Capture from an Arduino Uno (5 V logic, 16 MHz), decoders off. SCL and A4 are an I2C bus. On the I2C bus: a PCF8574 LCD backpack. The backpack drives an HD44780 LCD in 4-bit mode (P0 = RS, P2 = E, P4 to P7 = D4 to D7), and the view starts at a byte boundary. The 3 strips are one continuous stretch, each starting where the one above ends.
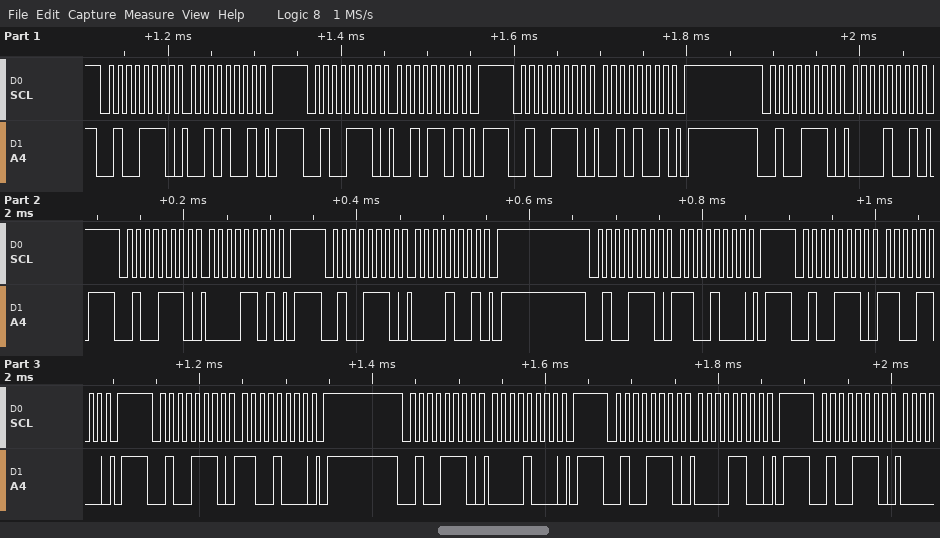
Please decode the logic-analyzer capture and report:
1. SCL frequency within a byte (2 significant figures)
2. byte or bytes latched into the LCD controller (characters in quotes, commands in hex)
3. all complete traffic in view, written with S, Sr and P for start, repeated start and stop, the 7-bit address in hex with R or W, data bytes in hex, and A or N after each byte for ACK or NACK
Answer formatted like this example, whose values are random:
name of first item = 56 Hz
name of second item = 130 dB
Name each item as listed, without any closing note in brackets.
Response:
SCL frequency within a byte = 100 kHz
byte or bytes latched into the LCD controller = ' '
all complete traffic in view, written with S, Sr and P for start, repeated start and stop, the 7-bit address in hex with R or W, data bytes in hex, and A or N after each byte for ACK or NACK = S 27W A 29 A P S 27W A 2D A P S 27W A 29 A P S 27W A 09 A P S 27W A 0D A P S 27W A 09 A P S 27W A C8 A P S 27W A CC A P S 27W A C8 A P S 27W A 08 A P S 27W A 0C A P S 27W A
